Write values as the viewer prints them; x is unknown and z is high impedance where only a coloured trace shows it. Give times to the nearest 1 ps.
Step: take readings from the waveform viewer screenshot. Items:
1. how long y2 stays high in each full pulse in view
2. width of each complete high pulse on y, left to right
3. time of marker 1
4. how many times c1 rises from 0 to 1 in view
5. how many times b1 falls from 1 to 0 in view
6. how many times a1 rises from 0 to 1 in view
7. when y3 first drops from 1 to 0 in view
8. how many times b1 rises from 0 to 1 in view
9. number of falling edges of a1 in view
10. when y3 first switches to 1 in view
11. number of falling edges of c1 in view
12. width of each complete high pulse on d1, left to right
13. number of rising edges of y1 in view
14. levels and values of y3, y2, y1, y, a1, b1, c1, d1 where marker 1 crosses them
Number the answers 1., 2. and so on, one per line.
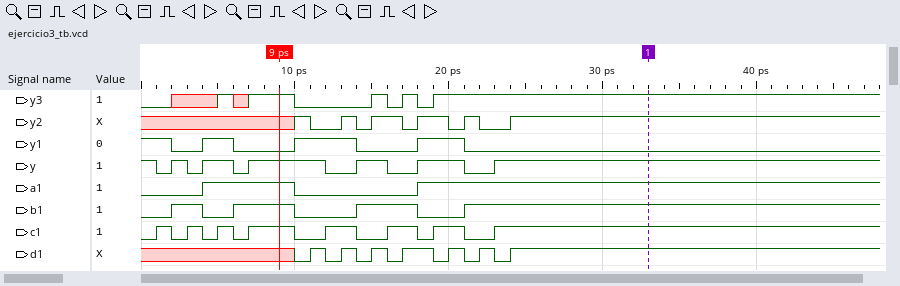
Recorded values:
1. 1 ps, 2 ps, 2 ps, 1 ps
2. 1 ps, 2 ps, 5 ps, 2 ps, 3 ps
3. 33 ps
4. 8
5. 3
6. 2
7. 10 ps
8. 4
9. 1
10. 5 ps
11. 7
12. 1 ps, 1 ps, 1 ps, 2 ps, 1 ps, 1 ps
13. 3
14. y3=1, y2=1, y1=0, y=1, a1=1, b1=1, c1=1, d1=1
